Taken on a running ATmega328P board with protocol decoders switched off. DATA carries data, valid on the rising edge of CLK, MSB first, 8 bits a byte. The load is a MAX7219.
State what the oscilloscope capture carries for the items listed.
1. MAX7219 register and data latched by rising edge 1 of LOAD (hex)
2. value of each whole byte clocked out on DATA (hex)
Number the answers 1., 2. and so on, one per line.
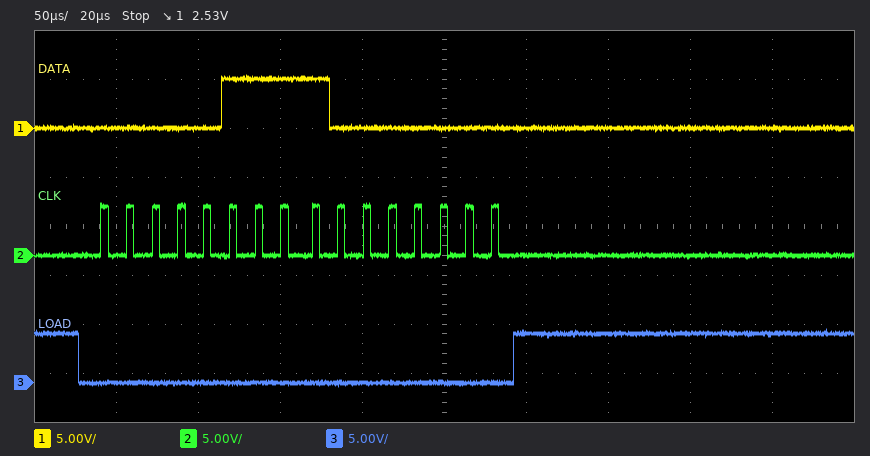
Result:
1. register 0x7, data 0x80
2. 07 80
